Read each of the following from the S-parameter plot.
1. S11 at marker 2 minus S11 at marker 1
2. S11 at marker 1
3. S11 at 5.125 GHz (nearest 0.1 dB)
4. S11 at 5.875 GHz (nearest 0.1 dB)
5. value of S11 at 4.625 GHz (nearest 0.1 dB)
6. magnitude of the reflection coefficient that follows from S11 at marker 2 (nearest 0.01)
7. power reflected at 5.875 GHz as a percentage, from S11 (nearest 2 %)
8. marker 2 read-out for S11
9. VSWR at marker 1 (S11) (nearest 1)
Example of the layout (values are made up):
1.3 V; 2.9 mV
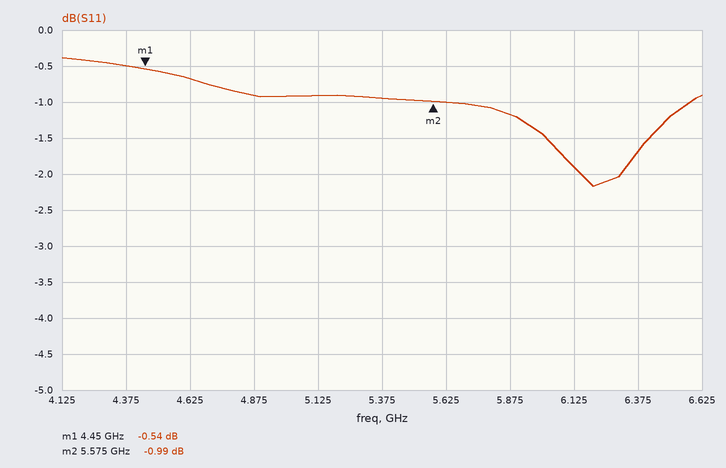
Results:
-0.45 dB; -0.54 dB; -0.9 dB; -1.2 dB; -0.7 dB; 0.89; 76 %; -0.99 dB; 32
